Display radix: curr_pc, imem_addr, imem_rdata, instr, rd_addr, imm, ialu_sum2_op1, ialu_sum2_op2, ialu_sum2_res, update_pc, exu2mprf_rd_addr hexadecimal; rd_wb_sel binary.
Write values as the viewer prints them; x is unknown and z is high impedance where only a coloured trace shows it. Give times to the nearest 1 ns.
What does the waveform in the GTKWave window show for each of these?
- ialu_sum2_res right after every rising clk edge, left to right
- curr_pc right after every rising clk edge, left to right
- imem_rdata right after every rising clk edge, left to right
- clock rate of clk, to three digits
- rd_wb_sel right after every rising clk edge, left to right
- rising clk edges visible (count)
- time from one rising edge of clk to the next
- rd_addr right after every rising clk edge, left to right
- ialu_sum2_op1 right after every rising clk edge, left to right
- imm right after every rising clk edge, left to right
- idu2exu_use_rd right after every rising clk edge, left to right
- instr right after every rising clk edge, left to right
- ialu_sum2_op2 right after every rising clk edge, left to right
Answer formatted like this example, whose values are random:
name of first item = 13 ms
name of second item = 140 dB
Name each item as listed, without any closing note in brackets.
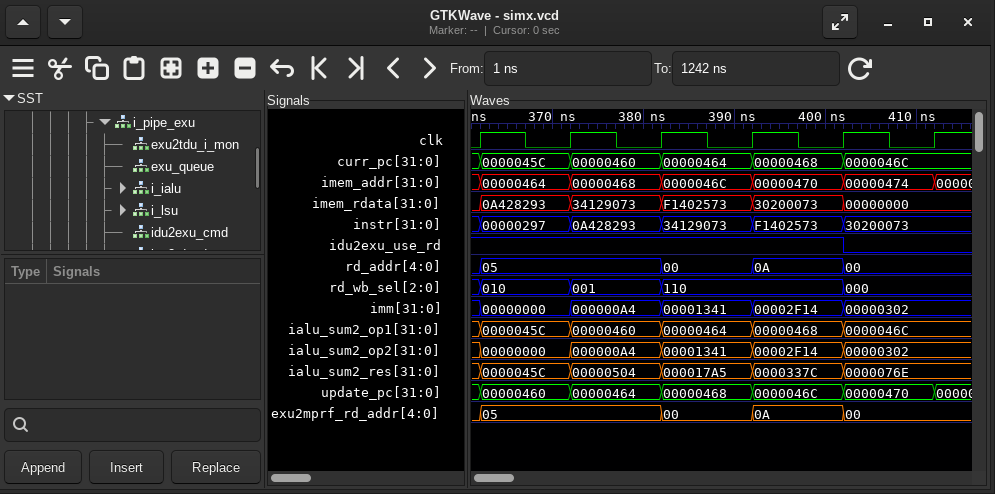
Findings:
ialu_sum2_res right after every rising clk edge, left to right = 0000045C, 00000504, 000017A5, 0000337C, 0000076E, 0000076E
curr_pc right after every rising clk edge, left to right = 0000045C, 00000460, 00000464, 00000468, 0000046C, 0000046C
imem_rdata right after every rising clk edge, left to right = 0A428293, 34129073, F1402573, 30200073, 00000000, 00000000
clock rate of clk, to three digits = 100 MHz
rd_wb_sel right after every rising clk edge, left to right = 010, 001, 110, 110, 000, 000
rising clk edges visible = 6
time from one rising edge of clk to the next = 10 ns
rd_addr right after every rising clk edge, left to right = 05, 05, 00, 0A, 00, 00
ialu_sum2_op1 right after every rising clk edge, left to right = 0000045C, 00000460, 00000464, 00000468, 0000046C, 0000046C
imm right after every rising clk edge, left to right = 00000000, 000000A4, 00001341, 00002F14, 00000302, 00000302
idu2exu_use_rd right after every rising clk edge, left to right = 1 1 1 1 0 0
instr right after every rising clk edge, left to right = 00000297, 0A428293, 34129073, F1402573, 30200073, 30200073
ialu_sum2_op2 right after every rising clk edge, left to right = 00000000, 000000A4, 00001341, 00002F14, 00000302, 00000302
